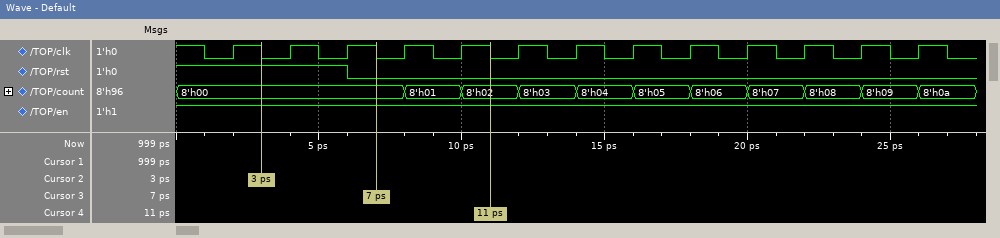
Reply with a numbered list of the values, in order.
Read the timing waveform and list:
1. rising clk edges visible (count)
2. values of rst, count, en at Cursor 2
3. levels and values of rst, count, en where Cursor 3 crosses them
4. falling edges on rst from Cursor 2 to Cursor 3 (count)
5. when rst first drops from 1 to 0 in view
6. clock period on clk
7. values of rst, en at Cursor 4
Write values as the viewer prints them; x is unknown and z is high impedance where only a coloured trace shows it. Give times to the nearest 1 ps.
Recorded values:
1. 13
2. rst=1, count=8'h00, en=1
3. rst=0, count=8'h00, en=1
4. 1
5. 6 ps
6. 2 ps
7. rst=0, en=1
